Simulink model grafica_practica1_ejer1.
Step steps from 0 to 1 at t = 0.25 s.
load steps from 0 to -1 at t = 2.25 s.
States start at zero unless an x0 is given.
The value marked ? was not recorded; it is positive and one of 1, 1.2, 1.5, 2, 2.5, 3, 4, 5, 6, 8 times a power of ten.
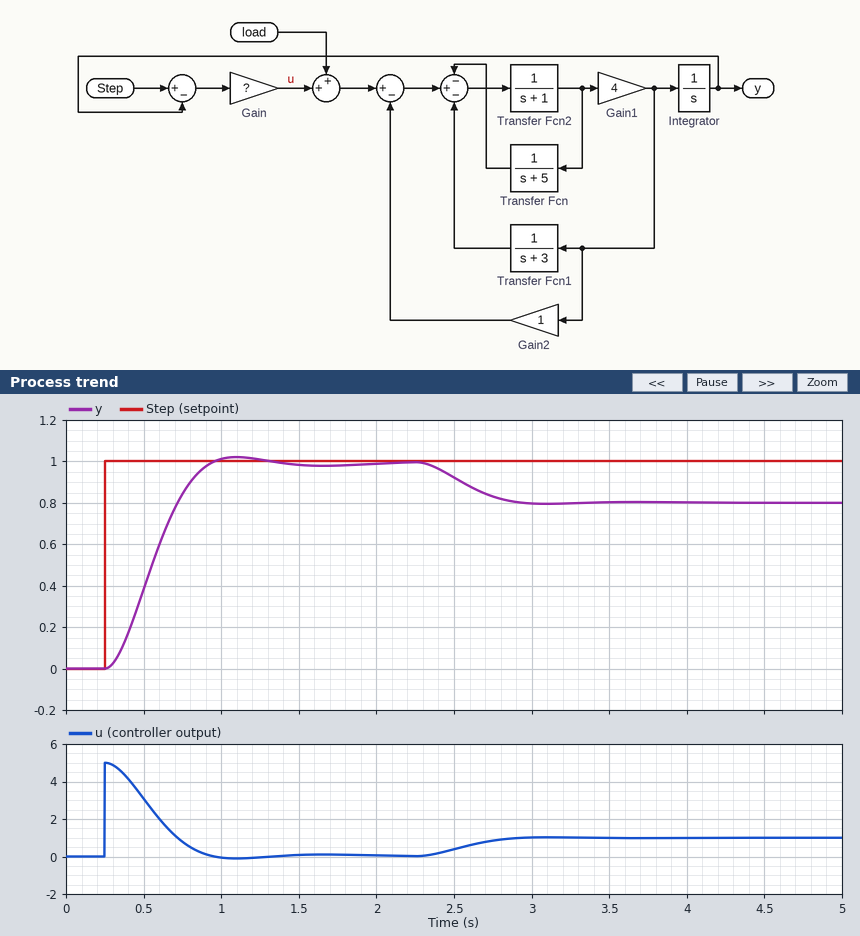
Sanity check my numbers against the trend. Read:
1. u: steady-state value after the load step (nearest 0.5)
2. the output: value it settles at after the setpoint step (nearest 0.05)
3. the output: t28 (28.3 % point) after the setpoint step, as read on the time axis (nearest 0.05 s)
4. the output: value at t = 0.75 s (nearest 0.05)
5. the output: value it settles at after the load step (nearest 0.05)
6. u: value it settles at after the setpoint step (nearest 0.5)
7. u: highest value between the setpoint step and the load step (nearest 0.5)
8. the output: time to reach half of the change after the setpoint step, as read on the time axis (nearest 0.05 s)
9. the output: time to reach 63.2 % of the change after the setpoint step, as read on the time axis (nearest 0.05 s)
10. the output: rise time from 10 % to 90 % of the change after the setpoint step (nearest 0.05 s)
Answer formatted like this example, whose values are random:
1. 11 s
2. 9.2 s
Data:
1. 1.0
2. 1.00
3. 0.45 s
4. 0.85
5. 0.80
6. 0.0
7. 5.0
8. 0.55 s
9. 0.60 s
10. 0.45 s
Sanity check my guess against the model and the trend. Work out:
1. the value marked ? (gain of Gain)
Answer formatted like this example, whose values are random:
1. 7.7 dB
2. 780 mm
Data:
1. 5
